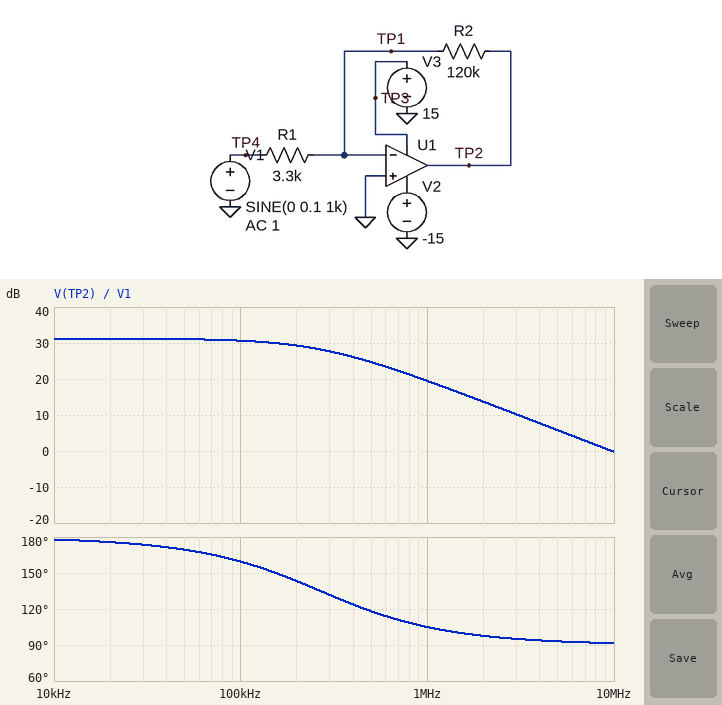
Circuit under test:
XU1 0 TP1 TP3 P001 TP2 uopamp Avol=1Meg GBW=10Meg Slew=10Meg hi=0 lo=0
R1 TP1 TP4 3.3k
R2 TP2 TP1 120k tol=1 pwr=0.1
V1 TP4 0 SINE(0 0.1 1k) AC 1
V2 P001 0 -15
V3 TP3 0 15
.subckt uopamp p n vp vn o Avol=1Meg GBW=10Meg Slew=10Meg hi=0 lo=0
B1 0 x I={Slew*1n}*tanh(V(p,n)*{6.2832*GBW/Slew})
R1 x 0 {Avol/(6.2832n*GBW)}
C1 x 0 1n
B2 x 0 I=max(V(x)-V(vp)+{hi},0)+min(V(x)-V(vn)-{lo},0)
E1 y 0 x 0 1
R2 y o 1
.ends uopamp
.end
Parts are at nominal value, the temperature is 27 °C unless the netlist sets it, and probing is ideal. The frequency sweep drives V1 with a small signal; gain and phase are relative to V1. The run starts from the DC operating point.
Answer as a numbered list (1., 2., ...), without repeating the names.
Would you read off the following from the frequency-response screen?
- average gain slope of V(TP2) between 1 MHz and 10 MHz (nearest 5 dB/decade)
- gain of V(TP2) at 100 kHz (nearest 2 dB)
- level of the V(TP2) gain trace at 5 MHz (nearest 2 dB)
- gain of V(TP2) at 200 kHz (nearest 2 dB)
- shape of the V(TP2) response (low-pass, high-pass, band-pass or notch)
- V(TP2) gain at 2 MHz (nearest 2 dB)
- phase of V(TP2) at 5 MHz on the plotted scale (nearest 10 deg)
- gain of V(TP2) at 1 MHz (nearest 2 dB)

1. -20 dB/decade
2. 30 dB
3. 6 dB
4. 30 dB
5. low-pass
6. 14 dB
7. 90 deg
8. 20 dB
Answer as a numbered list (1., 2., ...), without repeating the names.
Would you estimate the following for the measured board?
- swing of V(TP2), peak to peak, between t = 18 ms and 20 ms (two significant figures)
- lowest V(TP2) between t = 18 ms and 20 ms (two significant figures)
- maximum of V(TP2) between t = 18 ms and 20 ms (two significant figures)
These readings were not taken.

1. 7.3 V
2. -3.6 V
3. 3.6 V
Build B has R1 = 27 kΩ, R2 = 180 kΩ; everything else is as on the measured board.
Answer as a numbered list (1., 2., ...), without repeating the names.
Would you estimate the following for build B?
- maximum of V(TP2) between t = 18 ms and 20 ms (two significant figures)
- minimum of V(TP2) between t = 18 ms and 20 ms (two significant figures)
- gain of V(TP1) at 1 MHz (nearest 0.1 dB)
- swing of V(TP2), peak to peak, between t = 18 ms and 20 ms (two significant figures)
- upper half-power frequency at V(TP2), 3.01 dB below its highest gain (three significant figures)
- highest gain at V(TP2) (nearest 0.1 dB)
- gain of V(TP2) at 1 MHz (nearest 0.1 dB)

1. 670 mV
2. -670 mV
3. -5.5 dB
4. 1.3 V
5. 1.30 MHz
6. 16.5 dB
7. 14.5 dB
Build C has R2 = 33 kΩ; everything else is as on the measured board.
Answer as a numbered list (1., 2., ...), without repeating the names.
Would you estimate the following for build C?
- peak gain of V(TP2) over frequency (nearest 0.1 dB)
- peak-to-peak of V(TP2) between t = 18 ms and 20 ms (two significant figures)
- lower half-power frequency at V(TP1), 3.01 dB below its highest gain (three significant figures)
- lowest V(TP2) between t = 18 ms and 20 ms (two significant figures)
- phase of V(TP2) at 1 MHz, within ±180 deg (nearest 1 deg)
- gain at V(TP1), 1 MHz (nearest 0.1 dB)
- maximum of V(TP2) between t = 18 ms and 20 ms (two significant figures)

1. 20.0 dB
2. 2.0 V
3. 909 kHz
4. -1.0 V
5. 132 deg
6. -3.4 dB
7. 1.0 V
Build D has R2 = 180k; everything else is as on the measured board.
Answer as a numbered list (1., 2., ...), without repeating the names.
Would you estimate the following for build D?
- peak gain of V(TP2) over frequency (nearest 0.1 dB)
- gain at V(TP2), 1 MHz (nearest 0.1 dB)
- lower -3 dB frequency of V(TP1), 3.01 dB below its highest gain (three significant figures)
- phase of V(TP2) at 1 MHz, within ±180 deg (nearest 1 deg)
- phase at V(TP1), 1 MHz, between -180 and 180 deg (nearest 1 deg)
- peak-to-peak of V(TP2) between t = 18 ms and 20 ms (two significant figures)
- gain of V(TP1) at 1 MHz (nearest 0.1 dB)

1. 34.7 dB
2. 19.7 dB
3. 180 kHz
4. 100 deg
5. 10 deg
6. 11 V
7. -0.3 dB
